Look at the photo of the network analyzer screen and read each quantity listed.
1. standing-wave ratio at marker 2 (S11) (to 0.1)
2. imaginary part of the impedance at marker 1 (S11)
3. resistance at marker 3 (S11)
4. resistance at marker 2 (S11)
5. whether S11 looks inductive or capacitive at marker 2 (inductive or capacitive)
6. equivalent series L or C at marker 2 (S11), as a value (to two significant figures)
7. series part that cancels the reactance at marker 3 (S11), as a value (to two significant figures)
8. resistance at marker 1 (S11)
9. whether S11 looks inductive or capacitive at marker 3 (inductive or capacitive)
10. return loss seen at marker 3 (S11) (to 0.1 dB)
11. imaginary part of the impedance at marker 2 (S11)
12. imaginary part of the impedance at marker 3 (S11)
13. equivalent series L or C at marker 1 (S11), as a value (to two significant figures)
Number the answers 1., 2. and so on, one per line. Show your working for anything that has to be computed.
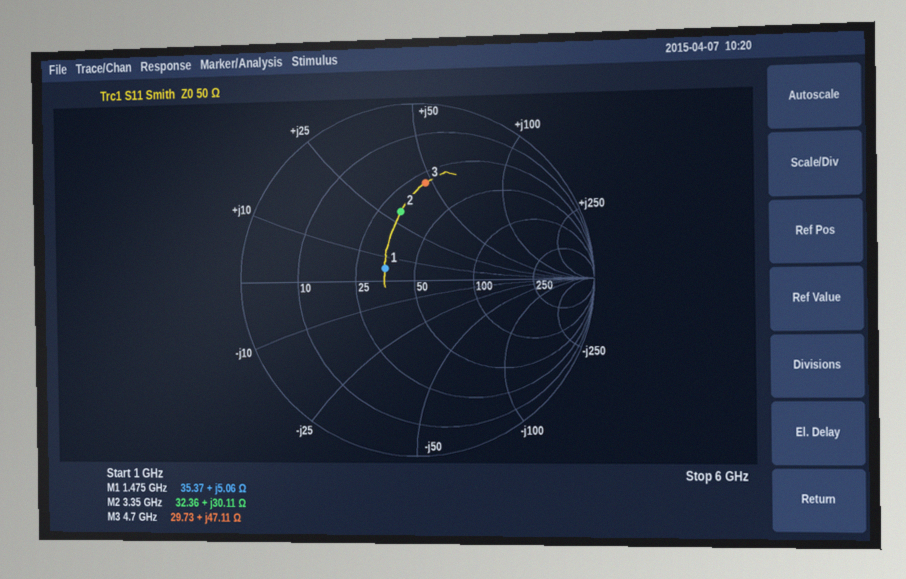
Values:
1. 2.3
2. +5.06 Ω
3. 29.73 Ω
4. 32.36 Ω
5. inductive
6. L = 30.11 Ω/(2π × 3.35 GHz) ≈ 1.4 nH
7. C = 1/(2π × 4.7 GHz × 47.11 Ω) ≈ 719 fF, so 720 fF to two significant figures
8. 35.37 Ω
9. inductive
10. 5.1 dB
11. +30.11 Ω
12. +47.11 Ω
13. L = 5.06 Ω/(2π × 1.475 GHz) ≈ 546 pH, so 550 pH to two significant figures
